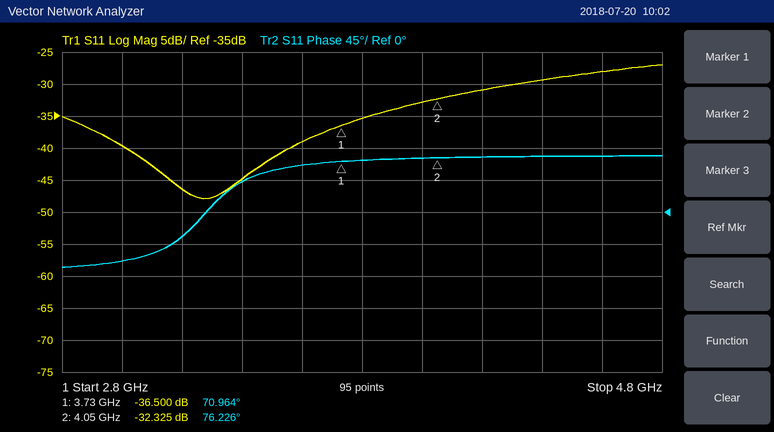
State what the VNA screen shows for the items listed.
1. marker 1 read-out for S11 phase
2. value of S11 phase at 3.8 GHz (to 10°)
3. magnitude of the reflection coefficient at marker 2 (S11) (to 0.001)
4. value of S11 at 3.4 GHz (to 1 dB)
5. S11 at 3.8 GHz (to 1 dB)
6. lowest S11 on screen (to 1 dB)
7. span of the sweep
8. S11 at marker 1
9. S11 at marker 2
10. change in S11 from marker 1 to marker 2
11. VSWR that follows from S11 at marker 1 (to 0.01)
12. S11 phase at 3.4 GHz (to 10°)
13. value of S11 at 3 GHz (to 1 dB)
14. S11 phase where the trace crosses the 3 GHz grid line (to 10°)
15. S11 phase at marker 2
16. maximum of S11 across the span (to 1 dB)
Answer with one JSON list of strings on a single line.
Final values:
["70.964°", "70°", "0.024", "-45 dB", "-35 dB", "-48 dB", "2 GHz", "-36.500 dB", "-32.325 dB", "4.175 dB", "1.03", "40°", "-40 dB", "-70°", "76.226°", "-27 dB"]
